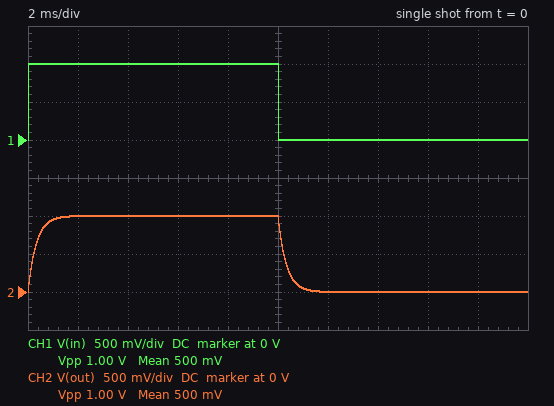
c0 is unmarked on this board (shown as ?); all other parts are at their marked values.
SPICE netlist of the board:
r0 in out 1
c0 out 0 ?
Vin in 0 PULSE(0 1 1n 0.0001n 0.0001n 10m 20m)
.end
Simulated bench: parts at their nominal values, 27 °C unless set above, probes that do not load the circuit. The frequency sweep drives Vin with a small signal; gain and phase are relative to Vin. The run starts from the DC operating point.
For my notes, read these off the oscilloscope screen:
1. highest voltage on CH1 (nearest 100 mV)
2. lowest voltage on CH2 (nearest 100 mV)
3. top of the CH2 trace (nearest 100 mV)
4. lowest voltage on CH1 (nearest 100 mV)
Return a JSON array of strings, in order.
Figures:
["1.0 V", "0 V", "1.0 V", "0 V"]
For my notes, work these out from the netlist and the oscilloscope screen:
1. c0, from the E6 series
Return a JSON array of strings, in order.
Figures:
["330 µF"]
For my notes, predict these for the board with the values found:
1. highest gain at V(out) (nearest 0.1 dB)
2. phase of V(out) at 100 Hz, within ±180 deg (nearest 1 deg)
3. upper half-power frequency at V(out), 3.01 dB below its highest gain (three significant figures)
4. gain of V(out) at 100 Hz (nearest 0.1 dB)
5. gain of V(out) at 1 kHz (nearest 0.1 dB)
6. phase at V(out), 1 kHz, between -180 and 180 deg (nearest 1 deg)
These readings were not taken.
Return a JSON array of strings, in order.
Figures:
["0 dB", "-12 deg", "482 Hz", "-0.2 dB", "-7.2 dB", "-64 deg"]
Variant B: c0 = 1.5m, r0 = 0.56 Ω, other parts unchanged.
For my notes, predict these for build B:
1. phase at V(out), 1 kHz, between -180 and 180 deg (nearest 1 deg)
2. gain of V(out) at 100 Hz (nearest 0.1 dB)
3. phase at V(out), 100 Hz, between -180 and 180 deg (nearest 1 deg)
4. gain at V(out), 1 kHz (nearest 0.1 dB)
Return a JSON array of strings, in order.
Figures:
["-79 deg", "-1.1 dB", "-28 deg", "-14.6 dB"]
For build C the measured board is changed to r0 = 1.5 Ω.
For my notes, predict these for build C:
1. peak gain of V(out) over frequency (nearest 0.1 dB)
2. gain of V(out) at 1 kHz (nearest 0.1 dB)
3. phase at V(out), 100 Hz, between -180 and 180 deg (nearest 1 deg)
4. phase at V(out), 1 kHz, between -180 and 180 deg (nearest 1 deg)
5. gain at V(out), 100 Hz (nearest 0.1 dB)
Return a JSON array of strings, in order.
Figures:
["0 dB", "-10.3 dB", "-17 deg", "-72 deg", "-0.4 dB"]
